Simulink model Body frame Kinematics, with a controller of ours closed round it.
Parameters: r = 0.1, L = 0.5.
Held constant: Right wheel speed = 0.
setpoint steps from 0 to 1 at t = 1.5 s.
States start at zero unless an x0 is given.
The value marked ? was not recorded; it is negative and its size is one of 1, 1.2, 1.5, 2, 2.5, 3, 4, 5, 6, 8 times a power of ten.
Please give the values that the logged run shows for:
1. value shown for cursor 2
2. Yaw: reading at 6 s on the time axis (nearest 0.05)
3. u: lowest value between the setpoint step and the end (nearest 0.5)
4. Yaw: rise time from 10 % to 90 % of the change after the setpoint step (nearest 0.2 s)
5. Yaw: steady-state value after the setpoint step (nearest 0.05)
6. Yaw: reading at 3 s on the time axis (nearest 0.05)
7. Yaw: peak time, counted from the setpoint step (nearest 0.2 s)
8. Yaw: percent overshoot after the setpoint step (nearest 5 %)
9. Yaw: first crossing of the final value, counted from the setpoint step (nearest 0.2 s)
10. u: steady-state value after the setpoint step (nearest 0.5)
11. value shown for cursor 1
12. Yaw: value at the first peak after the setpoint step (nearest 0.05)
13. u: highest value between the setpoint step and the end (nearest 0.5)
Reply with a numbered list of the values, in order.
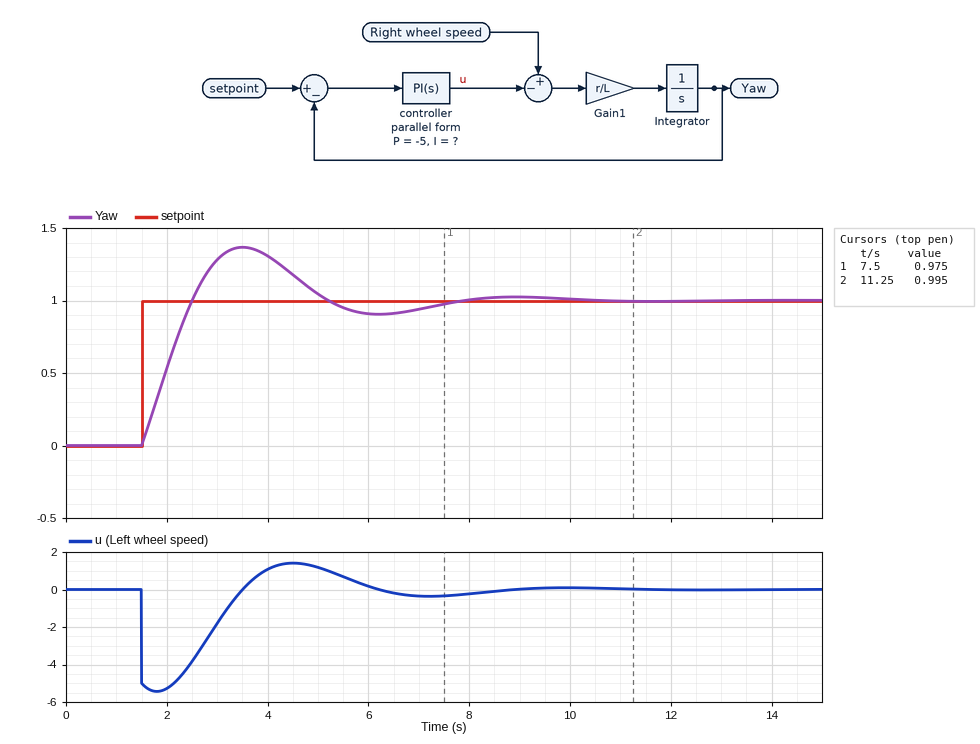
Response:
1. 0.995
2. 0.90
3. -5.5
4. 0.8 s
5. 1.00
6. 1.30
7. 2.0 s
8. 35 %
9. 1.0 s
10. 0.0
11. 0.975
12. 1.35
13. 1.5
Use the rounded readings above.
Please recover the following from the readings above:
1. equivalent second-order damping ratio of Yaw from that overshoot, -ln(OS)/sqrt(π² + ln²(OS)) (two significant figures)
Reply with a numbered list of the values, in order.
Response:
1. 0.32
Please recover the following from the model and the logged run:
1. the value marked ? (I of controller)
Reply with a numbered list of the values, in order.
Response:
1. -8
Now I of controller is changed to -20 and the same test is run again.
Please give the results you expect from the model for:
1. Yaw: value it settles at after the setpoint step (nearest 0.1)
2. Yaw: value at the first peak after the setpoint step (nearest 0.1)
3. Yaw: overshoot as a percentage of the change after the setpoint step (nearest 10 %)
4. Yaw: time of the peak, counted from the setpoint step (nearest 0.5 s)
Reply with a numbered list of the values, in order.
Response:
1. 1.0
2. 1.5
3. 50 %
4. 1.5 s
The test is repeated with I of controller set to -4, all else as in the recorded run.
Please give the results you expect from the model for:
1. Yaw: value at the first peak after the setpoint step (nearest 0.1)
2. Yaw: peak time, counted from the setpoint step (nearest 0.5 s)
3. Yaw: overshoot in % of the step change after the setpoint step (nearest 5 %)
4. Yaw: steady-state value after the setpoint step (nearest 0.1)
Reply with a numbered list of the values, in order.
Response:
1. 1.3
2. 2.5 s
3. 25 %
4. 1.0
